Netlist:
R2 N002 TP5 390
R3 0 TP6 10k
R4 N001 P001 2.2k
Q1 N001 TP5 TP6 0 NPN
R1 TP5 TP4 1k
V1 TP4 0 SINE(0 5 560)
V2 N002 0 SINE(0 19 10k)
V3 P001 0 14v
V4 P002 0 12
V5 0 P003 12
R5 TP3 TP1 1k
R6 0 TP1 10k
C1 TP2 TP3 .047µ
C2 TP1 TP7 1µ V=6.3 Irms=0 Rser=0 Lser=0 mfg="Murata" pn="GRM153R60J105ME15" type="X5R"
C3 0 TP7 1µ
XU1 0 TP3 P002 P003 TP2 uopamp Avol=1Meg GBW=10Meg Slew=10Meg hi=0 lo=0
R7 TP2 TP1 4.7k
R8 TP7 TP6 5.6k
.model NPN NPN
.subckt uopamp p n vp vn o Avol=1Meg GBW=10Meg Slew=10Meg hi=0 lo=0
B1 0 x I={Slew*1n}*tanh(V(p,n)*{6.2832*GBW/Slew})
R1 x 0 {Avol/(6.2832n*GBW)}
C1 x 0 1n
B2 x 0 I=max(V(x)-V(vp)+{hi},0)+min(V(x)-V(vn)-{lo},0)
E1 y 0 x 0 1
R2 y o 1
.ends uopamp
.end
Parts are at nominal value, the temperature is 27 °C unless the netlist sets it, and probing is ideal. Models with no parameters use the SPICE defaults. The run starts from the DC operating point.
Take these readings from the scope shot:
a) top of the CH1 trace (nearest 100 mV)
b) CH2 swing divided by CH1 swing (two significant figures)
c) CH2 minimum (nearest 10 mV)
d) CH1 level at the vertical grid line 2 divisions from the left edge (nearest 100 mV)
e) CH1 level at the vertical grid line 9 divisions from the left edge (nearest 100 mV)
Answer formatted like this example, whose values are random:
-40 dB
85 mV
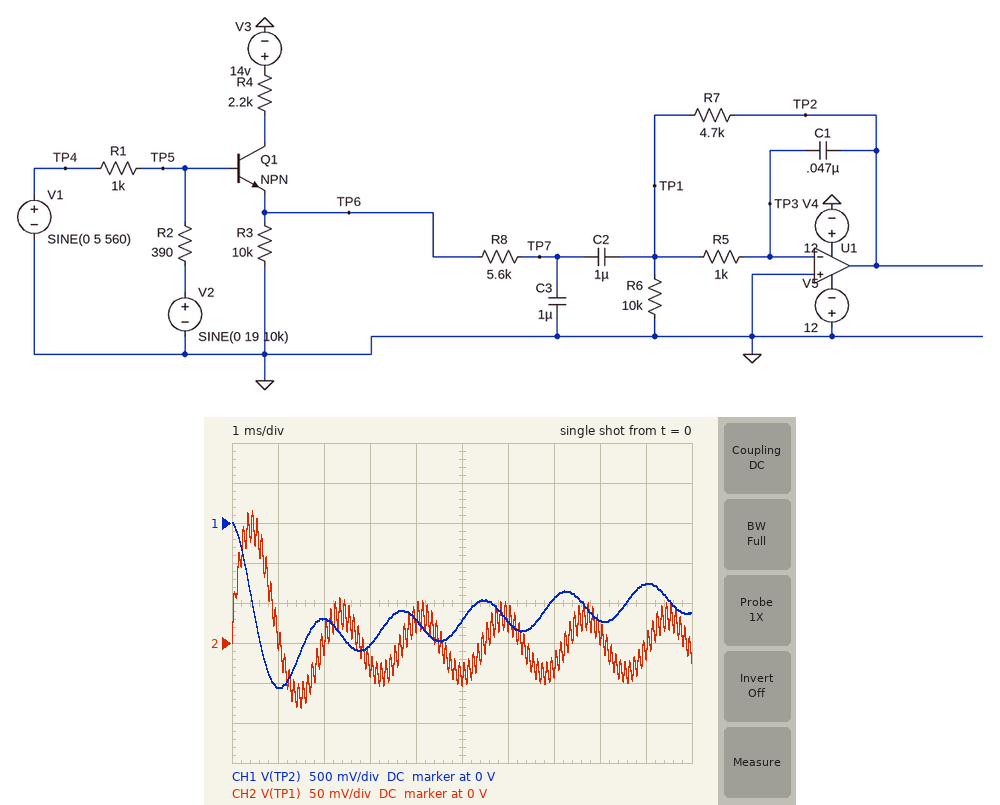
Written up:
0 V
0.12
-80 mV
-1.2 V
-800 mV
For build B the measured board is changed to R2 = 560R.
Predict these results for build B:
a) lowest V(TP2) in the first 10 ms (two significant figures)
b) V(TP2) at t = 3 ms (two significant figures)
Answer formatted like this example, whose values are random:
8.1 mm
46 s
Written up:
-1.9 V
-1.4 V
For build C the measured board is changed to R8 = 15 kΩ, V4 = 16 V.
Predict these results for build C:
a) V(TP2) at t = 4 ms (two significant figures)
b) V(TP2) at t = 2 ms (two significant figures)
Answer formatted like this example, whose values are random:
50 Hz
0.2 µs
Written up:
-520 mV
-490 mV
